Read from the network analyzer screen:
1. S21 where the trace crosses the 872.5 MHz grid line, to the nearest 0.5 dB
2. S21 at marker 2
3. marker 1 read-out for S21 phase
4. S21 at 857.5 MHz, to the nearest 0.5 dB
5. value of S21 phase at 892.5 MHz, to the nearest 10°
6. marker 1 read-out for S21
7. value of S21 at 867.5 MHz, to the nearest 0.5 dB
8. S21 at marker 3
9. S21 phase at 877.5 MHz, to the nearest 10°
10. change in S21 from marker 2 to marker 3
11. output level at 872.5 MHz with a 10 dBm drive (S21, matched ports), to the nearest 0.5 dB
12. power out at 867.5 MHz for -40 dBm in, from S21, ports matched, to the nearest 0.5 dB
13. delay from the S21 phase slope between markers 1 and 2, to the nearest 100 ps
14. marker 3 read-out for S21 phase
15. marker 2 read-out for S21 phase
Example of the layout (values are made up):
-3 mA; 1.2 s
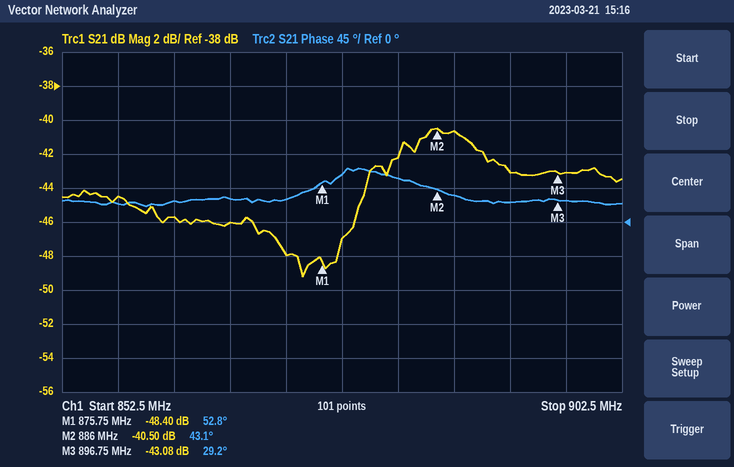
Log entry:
-48.0 dB; -40.50 dB; 52.8°; -44.5 dB; 30°; -48.40 dB; -46.0 dB; -43.08 dB; 60°; -2.58 dB; -38.0 dBm; -86.0 dBm; 2.6 ns; 29.2°; 43.1°
